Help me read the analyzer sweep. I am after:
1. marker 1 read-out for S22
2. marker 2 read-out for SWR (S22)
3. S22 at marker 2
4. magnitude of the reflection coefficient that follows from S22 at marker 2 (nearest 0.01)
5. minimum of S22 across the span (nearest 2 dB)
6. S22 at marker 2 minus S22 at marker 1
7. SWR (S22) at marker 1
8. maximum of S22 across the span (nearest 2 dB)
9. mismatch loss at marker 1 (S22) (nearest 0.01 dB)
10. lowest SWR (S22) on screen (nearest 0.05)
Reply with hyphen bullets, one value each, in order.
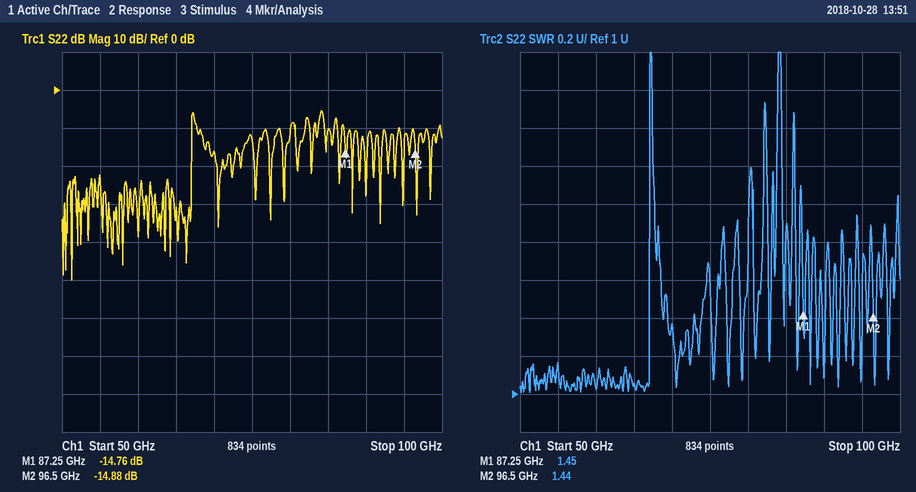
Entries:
- -14.76 dB
- 1.44
- -14.88 dB
- 0.18
- -50 dB
- -0.12 dB
- 1.45
- -6 dB
- 0.15 dB
- 1.00
